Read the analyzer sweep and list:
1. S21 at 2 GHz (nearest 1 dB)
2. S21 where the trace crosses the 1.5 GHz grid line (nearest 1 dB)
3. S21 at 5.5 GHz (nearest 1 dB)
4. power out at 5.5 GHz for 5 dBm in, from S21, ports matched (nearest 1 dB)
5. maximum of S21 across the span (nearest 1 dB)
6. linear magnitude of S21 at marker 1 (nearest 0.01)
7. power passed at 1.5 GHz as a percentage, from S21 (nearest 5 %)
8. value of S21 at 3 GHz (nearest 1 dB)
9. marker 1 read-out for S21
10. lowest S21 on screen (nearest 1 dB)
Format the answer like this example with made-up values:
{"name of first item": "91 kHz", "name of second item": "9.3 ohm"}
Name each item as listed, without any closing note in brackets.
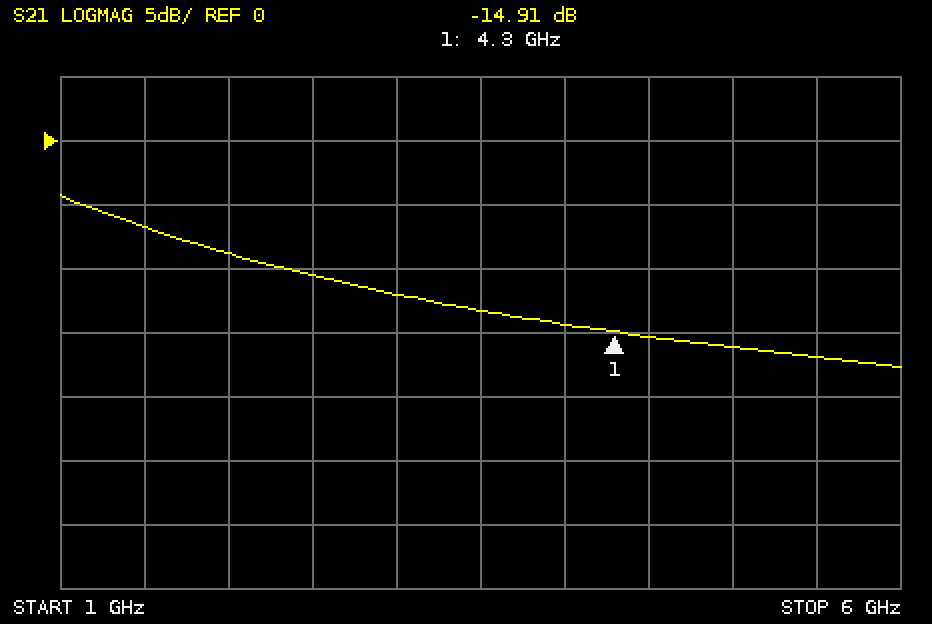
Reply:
{"S21 at 2 GHz": "-9 dB", "S21 where the trace crosses the 1.5 GHz grid line": "-7 dB", "S21 at 5.5 GHz": "-17 dB", "power out at 5.5 GHz for 5 dBm in, from S21, ports matched": "-12 dBm", "maximum of S21 across the span": "-4 dB", "linear magnitude of S21 at marker 1": "0.18", "power passed at 1.5 GHz as a percentage, from S21": "20 %", "value of S21 at 3 GHz": "-12 dB", "marker 1 read-out for S21": "-14.91 dB", "lowest S21 on screen": "-18 dB"}
